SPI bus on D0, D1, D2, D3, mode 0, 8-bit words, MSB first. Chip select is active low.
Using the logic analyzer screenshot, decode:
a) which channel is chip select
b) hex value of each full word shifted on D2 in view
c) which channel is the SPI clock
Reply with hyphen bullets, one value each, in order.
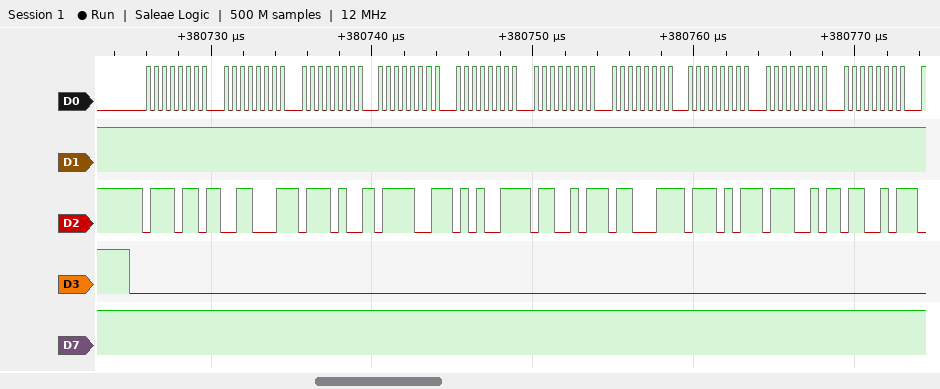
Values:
- D3
- 76, 31, 74, 79, 53, 65, 63, 75, 72, 65
- D0
